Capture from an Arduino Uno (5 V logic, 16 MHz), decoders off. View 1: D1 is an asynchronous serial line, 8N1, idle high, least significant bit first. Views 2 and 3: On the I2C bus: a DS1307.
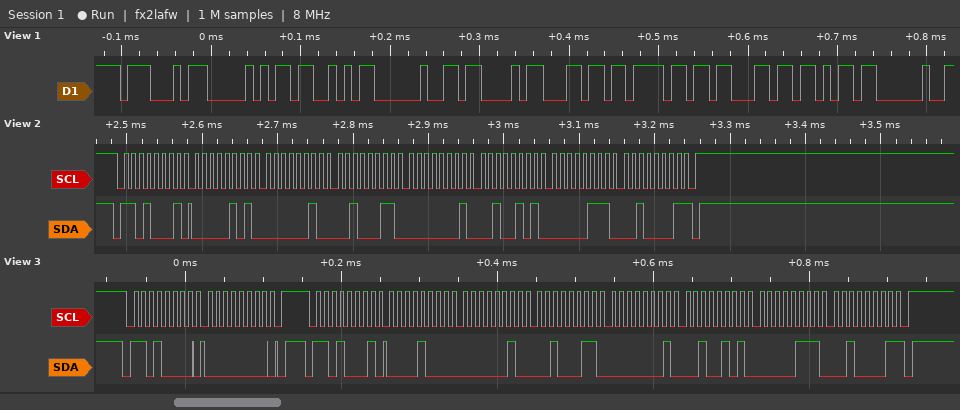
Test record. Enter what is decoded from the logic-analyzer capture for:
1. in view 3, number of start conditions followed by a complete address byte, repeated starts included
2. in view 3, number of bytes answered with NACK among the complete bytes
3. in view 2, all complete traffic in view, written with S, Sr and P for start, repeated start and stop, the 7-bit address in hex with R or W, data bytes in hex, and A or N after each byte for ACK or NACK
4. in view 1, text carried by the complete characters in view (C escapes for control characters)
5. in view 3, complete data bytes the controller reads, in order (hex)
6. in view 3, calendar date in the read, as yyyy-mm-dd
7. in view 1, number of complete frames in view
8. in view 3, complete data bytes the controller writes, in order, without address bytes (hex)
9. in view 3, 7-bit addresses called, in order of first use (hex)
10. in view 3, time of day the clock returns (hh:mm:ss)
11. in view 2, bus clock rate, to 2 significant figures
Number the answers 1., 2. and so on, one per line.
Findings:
1. 2
2. 1
3. S 68R A 05 A 02 A 23 A 01 A 25 A 07 A 21 N P
4. "GPS Clock "
5. 08 02 23 01 25 07 21
6. 2021-07-25
7. 10
8. 00
9. 0x68
10. 23:02:08
11. 100 kHz
